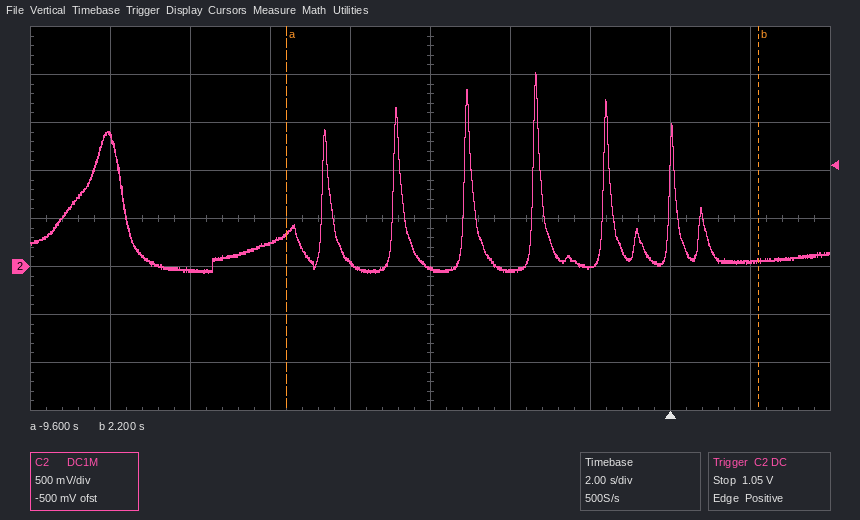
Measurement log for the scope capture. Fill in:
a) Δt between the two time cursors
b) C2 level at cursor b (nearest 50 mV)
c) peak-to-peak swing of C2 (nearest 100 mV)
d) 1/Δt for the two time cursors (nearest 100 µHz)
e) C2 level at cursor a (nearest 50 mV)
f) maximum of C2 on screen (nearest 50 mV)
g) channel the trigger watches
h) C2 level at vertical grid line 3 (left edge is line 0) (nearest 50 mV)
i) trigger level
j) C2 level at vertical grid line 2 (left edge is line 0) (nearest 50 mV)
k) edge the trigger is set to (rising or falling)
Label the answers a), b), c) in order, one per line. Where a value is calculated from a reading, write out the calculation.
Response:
a) 2.2 s − (-9.6 s) = 11.8 s
b) 50 mV
c) 2.10 V
d) 1 / 11.8 s ≈ 84.7 mHz
e) 350 mV
f) 2.00 V
g) C2
h) 250 mV
i) 1.05 V
j) -50 mV
k) rising
